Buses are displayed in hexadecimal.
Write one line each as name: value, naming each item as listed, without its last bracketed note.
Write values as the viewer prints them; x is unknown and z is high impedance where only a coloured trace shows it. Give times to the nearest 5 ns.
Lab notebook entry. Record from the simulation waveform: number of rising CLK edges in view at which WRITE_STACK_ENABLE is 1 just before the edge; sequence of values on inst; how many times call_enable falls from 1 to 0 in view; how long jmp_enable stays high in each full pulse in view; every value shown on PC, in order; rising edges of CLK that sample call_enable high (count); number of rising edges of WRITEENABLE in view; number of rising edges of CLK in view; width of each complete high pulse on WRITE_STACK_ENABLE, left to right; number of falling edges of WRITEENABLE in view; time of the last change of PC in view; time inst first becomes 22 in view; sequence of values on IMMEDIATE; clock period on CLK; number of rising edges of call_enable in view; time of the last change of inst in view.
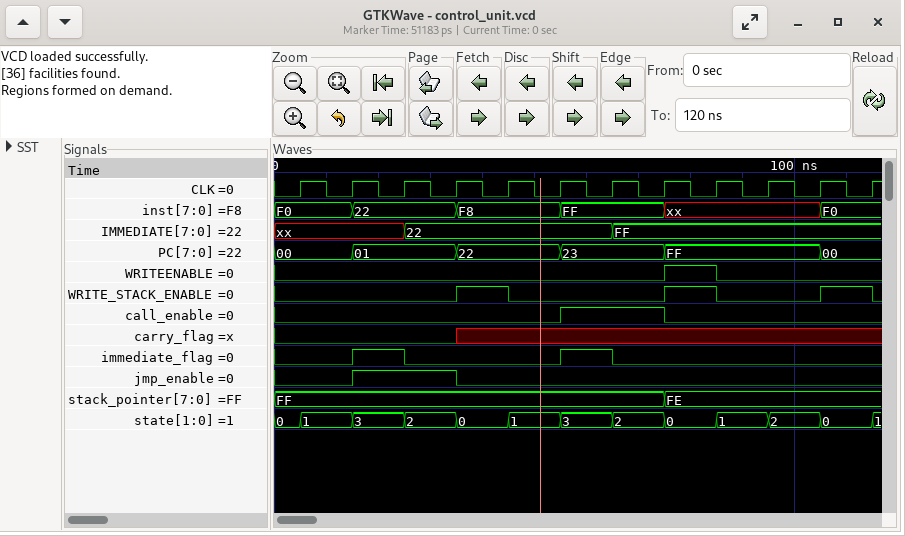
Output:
number of rising CLK edges in view at which WRITE_STACK_ENABLE is 1 just before the edge: 3
sequence of values on inst: F0, 22, F8, FF, xx, F0
how many times call_enable falls from 1 to 0 in view: 1
how long jmp_enable stays high in each full pulse in view: 20 ns
every value shown on PC, in order: 00, 01, 22, 23, FF, 00
rising edges of CLK that sample call_enable high: 2
number of rising edges of WRITEENABLE in view: 1
number of rising edges of CLK in view: 12
width of each complete high pulse on WRITE_STACK_ENABLE, left to right: 10 ns, 10 ns, 10 ns
number of falling edges of WRITEENABLE in view: 1
time of the last change of PC in view: 105 ns
time inst first becomes 22 in view: 15 ns
sequence of values on IMMEDIATE: xx, 22, FF
clock period on CLK: 10 ns
number of rising edges of call_enable in view: 1
time of the last change of inst in view: 105 ns
